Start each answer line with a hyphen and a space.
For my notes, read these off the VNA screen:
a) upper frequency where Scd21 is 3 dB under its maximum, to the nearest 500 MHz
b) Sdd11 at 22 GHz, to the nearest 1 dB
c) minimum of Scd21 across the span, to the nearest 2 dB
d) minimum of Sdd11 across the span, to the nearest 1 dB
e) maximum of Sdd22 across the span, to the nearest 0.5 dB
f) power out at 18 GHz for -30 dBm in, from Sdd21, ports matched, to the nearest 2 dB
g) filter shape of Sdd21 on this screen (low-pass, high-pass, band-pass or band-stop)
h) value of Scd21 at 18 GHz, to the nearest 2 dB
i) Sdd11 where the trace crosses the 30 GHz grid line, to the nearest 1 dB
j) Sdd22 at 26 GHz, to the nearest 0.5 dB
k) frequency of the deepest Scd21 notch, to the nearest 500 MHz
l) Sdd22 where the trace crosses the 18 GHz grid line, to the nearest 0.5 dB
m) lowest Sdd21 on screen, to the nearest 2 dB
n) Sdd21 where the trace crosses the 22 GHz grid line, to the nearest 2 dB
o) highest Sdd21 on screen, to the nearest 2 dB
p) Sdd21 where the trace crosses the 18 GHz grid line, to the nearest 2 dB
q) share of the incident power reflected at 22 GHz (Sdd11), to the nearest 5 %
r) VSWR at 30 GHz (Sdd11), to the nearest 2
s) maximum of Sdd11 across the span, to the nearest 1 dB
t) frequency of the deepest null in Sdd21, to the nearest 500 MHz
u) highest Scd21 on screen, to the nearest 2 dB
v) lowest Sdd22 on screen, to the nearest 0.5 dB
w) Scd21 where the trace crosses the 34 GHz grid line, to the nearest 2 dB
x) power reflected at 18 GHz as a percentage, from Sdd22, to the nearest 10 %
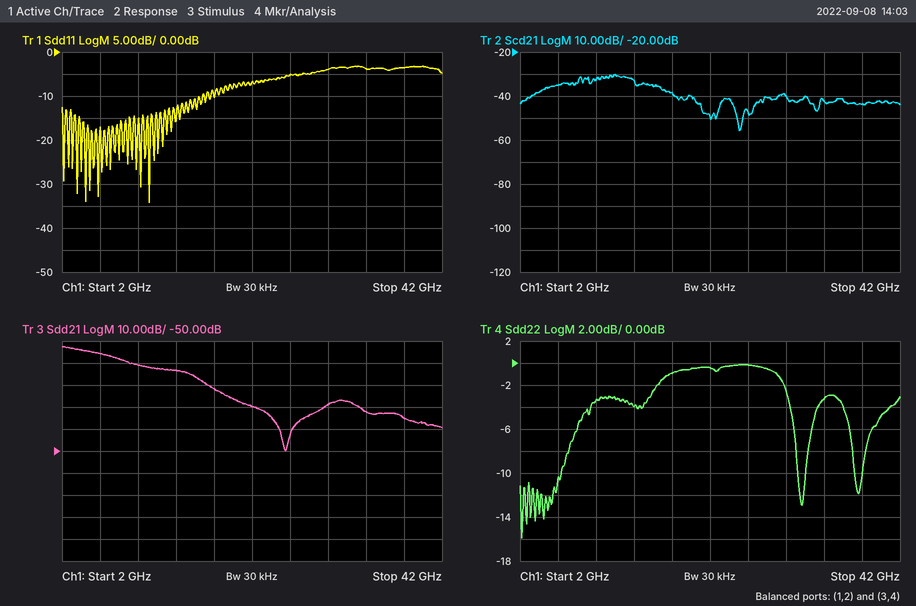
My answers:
- 14.0 GHz
- -7 dB
- -56 dB
- -34 dB
- 0.0 dB
- -52 dBm
- low-pass
- -38 dB
- -4 dB
- 0.0 dB
- 25.0 GHz
- -1.0 dB
- -50 dB
- -30 dB
- -2 dB
- -22 dB
- 20 %
- 4
- -3 dB
- 25.5 GHz
- -30 dB
- -16.0 dB
- -42 dB
- 80 %
